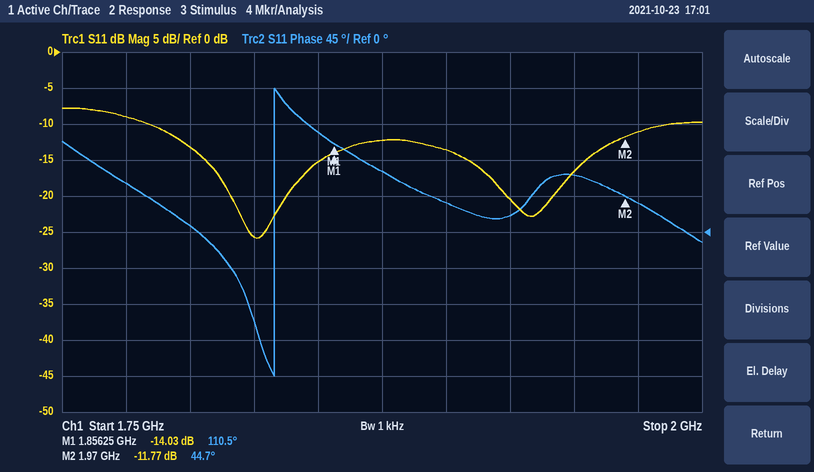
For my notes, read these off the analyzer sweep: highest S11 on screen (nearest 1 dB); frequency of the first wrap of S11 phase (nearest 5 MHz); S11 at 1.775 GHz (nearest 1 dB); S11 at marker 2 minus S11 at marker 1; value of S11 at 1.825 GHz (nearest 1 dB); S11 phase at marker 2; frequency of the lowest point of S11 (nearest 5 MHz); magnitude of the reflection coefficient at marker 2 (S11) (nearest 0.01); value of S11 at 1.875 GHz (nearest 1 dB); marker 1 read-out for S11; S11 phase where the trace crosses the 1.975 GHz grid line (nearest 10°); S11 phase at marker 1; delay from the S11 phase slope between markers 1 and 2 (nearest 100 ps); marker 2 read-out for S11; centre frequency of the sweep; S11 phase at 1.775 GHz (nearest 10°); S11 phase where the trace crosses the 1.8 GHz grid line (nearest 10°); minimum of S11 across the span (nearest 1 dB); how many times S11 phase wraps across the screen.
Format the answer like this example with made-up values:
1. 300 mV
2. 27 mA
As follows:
1. -8 dB
2. 1.835 GHz
3. -9 dB
4. 2.26 dB
5. -26 dB
6. 44.7°
7. 1.825 GHz
8. 0.26
9. -12 dB
10. -14.03 dB
11. 40°
12. 110.5°
13. 1.6 ns
14. -11.77 dB
15. 1.875 GHz
16. 60°
17. 10°
18. -26 dB
19. 1
